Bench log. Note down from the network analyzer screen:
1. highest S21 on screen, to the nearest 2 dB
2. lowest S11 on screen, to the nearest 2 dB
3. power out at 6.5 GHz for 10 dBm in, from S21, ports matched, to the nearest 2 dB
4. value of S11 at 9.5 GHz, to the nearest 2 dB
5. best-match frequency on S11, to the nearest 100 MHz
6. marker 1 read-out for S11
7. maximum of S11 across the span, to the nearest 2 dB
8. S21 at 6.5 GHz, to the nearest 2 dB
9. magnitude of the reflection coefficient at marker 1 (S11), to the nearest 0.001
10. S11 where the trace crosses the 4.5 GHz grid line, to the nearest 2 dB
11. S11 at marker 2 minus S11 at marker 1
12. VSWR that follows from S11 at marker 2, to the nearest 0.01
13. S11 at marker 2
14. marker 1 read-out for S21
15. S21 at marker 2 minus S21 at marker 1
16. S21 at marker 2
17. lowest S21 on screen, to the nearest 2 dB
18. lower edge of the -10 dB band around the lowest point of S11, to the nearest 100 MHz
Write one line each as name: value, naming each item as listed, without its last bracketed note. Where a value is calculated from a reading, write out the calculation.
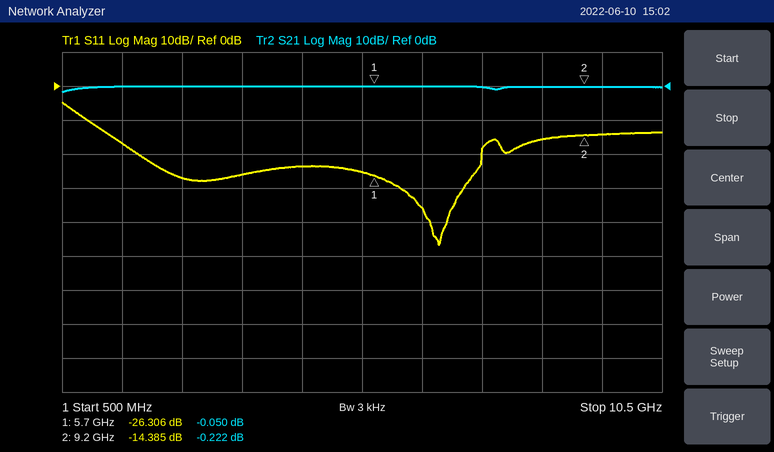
highest S21 on screen, to the nearest 2 dB: 0 dB
lowest S11 on screen, to the nearest 2 dB: -46 dB
power out at 6.5 GHz for 10 dBm in, from S21, ports matched, to the nearest 2 dB: 10 dBm + (0 dB) = 10 dBm
value of S11 at 9.5 GHz, to the nearest 2 dB: -14 dB
best-match frequency on S11, to the nearest 100 MHz: 6.8 GHz
marker 1 read-out for S11: -26.306 dB
maximum of S11 across the span, to the nearest 2 dB: -4 dB
S21 at 6.5 GHz, to the nearest 2 dB: 0 dB
magnitude of the reflection coefficient at marker 1 (S11), to the nearest 0.001: 10^(-26.306/20) ≈ 0.048
S11 where the trace crosses the 4.5 GHz grid line, to the nearest 2 dB: -24 dB
S11 at marker 2 minus S11 at marker 1: -14.385 − (-26.306) = 11.921 dB
VSWR that follows from S11 at marker 2, to the nearest 0.01: (1 + 0.1909)/(1 − 0.1909) ≈ 1.47
S11 at marker 2: -14.385 dB
marker 1 read-out for S21: -0.050 dB
S21 at marker 2 minus S21 at marker 1: -0.222 − (-0.05) = -0.172 dB
S21 at marker 2: -0.222 dB
lowest S21 on screen, to the nearest 2 dB: -2 dB
lower edge of the -10 dB band around the lowest point of S11, to the nearest 100 MHz: 900 MHz
